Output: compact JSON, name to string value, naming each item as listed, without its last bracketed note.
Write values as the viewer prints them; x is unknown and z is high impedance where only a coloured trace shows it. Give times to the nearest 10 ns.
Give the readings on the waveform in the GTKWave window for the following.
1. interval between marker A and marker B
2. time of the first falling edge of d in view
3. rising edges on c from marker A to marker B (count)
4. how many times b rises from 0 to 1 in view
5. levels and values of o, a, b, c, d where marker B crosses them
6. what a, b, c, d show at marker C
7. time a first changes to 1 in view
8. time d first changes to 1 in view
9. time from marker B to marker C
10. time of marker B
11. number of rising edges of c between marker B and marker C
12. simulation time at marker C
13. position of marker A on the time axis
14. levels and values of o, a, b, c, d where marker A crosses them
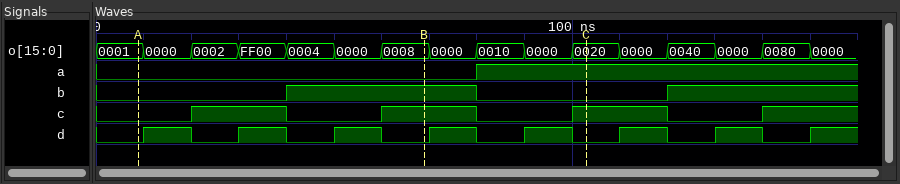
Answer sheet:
{"interval between marker A and marker B": "60 ns", "time of the first falling edge of d in view": "20 ns", "rising edges on c from marker A to marker B": "2", "how many times b rises from 0 to 1 in view": "2", "levels and values of o, a, b, c, d where marker B crosses them": "o=0008, a=0, b=1, c=1, d=0", "what a, b, c, d show at marker C": "a=1, b=0, c=1, d=0", "time a first changes to 1 in view": "80 ns", "time d first changes to 1 in view": "10 ns", "time from marker B to marker C": "30 ns", "time of marker B": "70 ns", "number of rising edges of c between marker B and marker C": "1", "simulation time at marker C": "100 ns", "position of marker A on the time axis": "10 ns", "levels and values of o, a, b, c, d where marker A crosses them": "o=0001, a=0, b=0, c=0, d=0"}
